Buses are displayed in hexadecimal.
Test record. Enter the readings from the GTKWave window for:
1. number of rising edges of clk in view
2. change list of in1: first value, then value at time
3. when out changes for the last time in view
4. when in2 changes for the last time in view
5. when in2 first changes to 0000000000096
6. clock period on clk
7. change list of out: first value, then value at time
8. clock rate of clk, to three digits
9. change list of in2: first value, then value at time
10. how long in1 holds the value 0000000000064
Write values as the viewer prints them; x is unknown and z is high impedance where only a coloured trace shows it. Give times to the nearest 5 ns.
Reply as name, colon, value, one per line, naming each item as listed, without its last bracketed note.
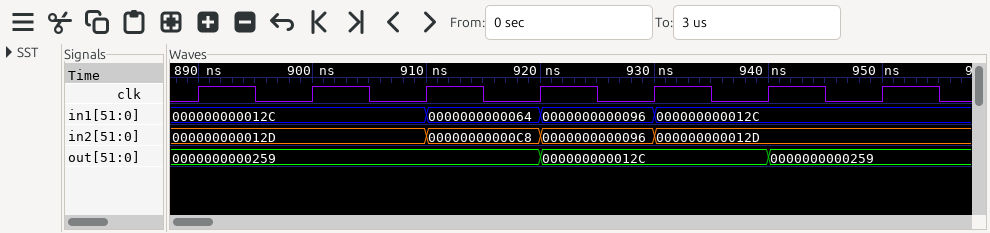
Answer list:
number of rising edges of clk in view: 7
change list of in1: first value, then value at time: 000000000012C, 0000000000064 at 910 ns, 0000000000096 at 920 ns, 000000000012C at 930 ns
when out changes for the last time in view: 940 ns
when in2 changes for the last time in view: 930 ns
when in2 first changes to 0000000000096: 920 ns
clock period on clk: 10 ns
change list of out: first value, then value at time: 0000000000259, 000000000012C at 920 ns, 0000000000259 at 940 ns
clock rate of clk, to three digits: 100 MHz
change list of in2: first value, then value at time: 000000000012D, 00000000000C8 at 910 ns, 0000000000096 at 920 ns, 000000000012D at 930 ns
how long in1 holds the value 0000000000064: 10 ns
